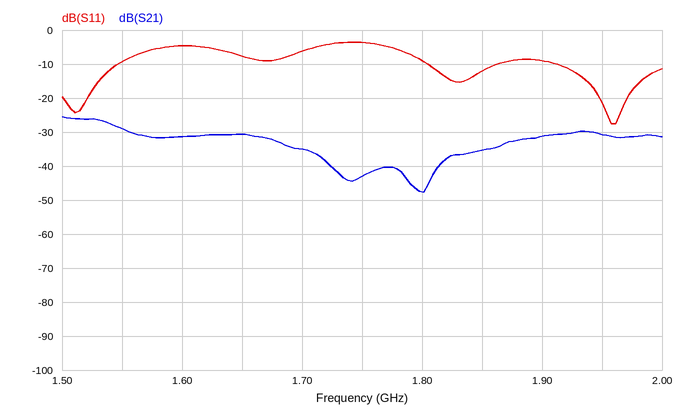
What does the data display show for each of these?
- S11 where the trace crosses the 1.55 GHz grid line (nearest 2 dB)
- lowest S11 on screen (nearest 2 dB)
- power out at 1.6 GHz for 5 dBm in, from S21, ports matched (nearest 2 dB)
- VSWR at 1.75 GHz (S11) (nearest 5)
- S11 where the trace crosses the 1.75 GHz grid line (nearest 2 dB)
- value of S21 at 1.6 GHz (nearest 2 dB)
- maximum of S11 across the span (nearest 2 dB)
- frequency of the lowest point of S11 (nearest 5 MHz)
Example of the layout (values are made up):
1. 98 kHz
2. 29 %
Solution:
1. -10 dB
2. -28 dB
3. -26 dBm
4. 5
5. -4 dB
6. -32 dB
7. -4 dB
8. 1.960 GHz
